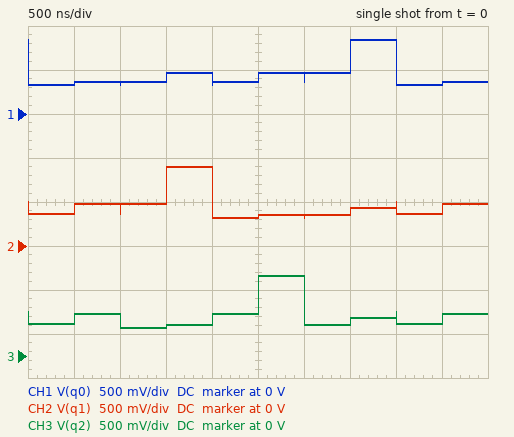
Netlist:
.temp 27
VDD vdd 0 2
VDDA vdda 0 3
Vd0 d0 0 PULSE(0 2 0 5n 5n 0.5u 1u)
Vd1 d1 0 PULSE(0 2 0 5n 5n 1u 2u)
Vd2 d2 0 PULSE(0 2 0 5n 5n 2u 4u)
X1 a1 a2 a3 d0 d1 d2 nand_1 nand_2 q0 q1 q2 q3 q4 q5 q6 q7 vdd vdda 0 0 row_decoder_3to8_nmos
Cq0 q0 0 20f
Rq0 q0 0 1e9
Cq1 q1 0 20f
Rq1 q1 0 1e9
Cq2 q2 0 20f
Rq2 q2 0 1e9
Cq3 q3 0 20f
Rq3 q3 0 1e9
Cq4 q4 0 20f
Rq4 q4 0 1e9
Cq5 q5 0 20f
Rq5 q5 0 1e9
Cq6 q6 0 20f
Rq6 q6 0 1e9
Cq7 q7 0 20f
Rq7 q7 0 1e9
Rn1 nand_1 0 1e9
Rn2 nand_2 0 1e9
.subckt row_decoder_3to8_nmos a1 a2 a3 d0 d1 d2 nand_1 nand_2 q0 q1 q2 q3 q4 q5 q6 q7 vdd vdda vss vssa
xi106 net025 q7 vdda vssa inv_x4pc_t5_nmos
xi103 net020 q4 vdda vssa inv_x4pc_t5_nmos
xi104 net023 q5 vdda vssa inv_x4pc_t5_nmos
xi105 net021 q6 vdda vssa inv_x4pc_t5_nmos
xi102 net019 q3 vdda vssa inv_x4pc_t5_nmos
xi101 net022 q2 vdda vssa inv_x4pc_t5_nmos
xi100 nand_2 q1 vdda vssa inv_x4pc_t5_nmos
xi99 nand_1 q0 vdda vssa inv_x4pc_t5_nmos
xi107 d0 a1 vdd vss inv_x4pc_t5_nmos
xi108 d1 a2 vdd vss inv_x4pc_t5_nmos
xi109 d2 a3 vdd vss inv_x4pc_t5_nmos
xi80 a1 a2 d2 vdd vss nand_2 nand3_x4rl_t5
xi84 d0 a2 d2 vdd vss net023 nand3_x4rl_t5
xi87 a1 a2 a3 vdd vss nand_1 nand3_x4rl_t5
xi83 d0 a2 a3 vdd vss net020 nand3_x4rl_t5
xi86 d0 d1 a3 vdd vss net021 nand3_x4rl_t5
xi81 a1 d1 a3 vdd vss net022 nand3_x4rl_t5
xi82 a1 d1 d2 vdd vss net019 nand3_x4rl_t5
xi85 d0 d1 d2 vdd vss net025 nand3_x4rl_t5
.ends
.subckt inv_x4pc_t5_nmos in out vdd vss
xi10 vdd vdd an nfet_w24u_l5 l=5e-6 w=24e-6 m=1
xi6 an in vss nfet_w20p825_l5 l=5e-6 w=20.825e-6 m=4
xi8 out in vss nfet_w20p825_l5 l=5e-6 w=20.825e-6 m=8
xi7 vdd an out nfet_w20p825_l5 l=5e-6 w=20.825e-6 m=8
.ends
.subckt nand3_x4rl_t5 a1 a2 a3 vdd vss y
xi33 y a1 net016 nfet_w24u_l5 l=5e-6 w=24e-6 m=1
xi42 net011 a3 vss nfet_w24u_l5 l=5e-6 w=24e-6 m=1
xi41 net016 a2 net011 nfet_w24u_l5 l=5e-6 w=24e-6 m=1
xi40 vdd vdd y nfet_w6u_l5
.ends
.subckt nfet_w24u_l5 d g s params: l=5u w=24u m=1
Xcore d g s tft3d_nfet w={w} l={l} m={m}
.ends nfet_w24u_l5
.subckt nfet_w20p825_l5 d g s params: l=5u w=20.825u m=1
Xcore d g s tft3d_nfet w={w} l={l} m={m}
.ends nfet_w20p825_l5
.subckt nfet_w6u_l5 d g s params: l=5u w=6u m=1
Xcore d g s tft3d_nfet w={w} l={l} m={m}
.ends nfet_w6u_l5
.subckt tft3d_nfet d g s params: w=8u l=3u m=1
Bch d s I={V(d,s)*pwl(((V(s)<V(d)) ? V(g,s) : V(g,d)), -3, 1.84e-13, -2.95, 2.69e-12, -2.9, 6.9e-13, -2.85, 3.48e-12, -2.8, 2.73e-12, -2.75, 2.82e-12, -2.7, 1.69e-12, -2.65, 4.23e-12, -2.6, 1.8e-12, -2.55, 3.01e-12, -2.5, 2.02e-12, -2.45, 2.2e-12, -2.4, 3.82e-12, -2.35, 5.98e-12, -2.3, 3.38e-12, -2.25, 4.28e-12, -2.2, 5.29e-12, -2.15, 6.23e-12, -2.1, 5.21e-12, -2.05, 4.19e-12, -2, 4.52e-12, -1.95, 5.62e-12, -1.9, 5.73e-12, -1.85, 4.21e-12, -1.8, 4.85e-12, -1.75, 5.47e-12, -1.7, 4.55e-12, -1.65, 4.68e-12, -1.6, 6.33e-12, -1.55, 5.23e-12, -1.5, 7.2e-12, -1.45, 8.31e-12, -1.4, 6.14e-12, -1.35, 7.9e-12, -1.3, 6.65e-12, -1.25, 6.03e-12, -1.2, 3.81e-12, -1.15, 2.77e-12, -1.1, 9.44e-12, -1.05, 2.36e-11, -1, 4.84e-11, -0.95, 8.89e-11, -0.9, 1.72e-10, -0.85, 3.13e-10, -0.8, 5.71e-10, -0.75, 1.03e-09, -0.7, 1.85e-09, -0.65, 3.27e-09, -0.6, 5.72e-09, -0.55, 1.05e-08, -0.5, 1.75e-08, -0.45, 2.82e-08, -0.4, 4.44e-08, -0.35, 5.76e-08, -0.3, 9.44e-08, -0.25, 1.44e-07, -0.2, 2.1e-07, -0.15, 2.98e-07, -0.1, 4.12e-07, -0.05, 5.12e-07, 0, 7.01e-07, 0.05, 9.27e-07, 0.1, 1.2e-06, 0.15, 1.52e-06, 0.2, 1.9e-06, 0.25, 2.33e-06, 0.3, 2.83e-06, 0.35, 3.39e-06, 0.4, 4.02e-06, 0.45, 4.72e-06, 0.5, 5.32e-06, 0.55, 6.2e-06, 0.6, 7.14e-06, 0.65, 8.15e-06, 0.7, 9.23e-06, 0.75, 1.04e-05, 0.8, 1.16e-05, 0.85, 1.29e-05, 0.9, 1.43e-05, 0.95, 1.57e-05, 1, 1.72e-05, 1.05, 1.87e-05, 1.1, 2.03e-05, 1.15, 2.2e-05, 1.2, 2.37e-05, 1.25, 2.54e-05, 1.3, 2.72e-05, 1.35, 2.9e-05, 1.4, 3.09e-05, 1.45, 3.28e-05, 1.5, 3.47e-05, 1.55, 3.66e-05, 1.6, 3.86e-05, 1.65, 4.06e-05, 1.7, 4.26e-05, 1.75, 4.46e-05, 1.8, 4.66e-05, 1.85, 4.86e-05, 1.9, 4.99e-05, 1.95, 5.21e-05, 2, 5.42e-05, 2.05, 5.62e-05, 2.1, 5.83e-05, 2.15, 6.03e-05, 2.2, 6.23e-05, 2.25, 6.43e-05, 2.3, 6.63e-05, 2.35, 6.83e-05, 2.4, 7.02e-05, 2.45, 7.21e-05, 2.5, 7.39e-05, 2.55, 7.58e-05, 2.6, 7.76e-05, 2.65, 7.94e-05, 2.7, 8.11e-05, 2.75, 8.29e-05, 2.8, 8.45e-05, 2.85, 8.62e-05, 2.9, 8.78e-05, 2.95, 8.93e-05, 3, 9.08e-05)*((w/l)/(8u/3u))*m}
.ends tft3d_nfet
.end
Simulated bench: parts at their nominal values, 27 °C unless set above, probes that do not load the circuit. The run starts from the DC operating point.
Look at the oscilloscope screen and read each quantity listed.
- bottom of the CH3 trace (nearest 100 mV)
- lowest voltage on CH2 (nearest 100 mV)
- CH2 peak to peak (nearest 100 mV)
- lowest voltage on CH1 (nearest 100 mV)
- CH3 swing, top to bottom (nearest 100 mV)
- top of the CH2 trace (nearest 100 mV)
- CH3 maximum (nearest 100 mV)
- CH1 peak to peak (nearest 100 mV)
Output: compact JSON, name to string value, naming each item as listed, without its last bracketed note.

{"bottom of the CH3 trace": "300 mV", "lowest voltage on CH2": "300 mV", "CH2 peak to peak": "600 mV", "lowest voltage on CH1": "300 mV", "CH3 swing, top to bottom": "600 mV", "top of the CH2 trace": "900 mV", "CH3 maximum": "900 mV", "CH1 peak to peak": "500 mV"}
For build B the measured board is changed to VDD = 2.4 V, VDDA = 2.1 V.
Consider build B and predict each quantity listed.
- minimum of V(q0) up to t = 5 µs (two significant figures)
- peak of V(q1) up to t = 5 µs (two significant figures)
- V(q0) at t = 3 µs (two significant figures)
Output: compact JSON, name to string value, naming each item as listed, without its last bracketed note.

{"minimum of V(q0) up to t = 5 µs": "91 mV", "peak of V(q1) up to t = 5 µs": "350 mV", "V(q0) at t = 3 µs": "140 mV"}
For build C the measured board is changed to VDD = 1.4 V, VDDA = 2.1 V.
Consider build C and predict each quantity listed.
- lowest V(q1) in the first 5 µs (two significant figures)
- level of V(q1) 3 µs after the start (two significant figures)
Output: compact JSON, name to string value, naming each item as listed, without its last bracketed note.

{"lowest V(q1) in the first 5 µs": "260 mV", "level of V(q1) 3 µs after the start": "290 mV"}
